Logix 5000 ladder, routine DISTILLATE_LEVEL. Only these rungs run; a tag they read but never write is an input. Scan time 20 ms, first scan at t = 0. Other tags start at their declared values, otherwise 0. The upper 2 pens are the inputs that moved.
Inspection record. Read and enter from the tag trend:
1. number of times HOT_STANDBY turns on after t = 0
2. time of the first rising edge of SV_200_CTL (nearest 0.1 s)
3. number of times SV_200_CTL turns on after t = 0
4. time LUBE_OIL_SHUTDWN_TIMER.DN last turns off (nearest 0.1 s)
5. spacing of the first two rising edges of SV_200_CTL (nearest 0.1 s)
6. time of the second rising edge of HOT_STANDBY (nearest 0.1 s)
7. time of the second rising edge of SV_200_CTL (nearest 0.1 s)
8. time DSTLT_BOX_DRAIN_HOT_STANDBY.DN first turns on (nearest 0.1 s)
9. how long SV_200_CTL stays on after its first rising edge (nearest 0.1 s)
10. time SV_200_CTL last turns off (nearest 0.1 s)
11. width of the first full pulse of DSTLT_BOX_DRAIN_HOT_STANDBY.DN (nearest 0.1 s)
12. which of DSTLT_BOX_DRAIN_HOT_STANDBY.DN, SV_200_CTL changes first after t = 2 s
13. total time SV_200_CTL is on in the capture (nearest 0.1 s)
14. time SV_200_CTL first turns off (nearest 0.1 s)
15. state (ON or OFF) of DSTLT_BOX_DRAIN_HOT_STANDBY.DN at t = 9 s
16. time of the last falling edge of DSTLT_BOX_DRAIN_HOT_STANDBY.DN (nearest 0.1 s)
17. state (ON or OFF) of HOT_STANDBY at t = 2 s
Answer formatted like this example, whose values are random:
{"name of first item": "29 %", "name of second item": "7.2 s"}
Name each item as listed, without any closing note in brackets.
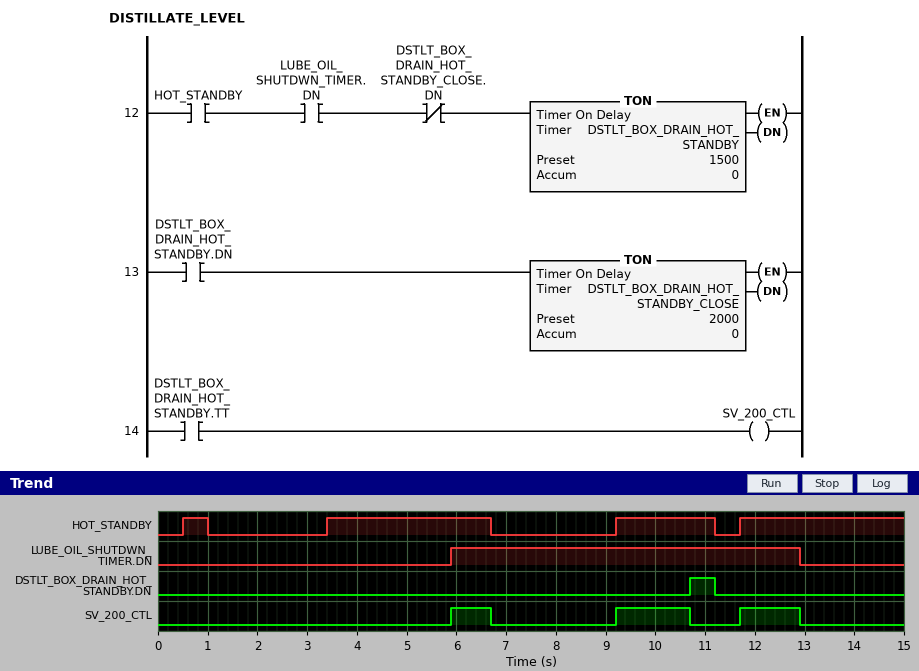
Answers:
{"number of times HOT_STANDBY turns on after t = 0": "4", "time of the first rising edge of SV_200_CTL": "5.9 s", "number of times SV_200_CTL turns on after t = 0": "3", "time LUBE_OIL_SHUTDWN_TIMER.DN last turns off": "12.9 s", "spacing of the first two rising edges of SV_200_CTL": "3.3 s", "time of the second rising edge of HOT_STANDBY": "3.4 s", "time of the second rising edge of SV_200_CTL": "9.2 s", "time DSTLT_BOX_DRAIN_HOT_STANDBY.DN first turns on": "10.7 s", "how long SV_200_CTL stays on after its first rising edge": "0.8 s", "time SV_200_CTL last turns off": "12.9 s", "width of the first full pulse of DSTLT_BOX_DRAIN_HOT_STANDBY.DN": "0.5 s", "which of DSTLT_BOX_DRAIN_HOT_STANDBY.DN, SV_200_CTL changes first after t = 2 s": "SV_200_CTL", "total time SV_200_CTL is on in the capture": "3.5 s", "time SV_200_CTL first turns off": "6.7 s", "state (ON or OFF) of DSTLT_BOX_DRAIN_HOT_STANDBY.DN at t = 9 s": "OFF", "time of the last falling edge of DSTLT_BOX_DRAIN_HOT_STANDBY.DN": "11.2 s", "state (ON or OFF) of HOT_STANDBY at t = 2 s": "OFF"}
